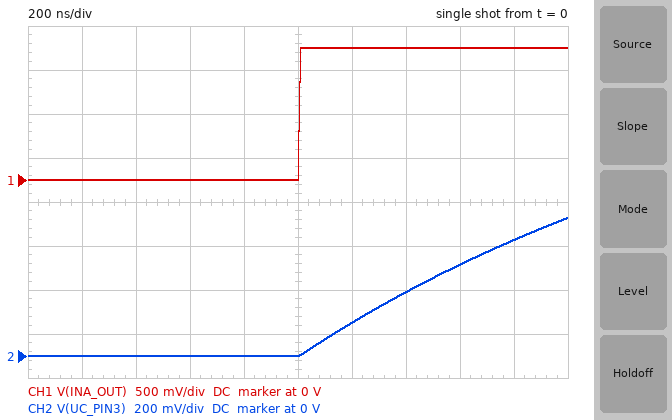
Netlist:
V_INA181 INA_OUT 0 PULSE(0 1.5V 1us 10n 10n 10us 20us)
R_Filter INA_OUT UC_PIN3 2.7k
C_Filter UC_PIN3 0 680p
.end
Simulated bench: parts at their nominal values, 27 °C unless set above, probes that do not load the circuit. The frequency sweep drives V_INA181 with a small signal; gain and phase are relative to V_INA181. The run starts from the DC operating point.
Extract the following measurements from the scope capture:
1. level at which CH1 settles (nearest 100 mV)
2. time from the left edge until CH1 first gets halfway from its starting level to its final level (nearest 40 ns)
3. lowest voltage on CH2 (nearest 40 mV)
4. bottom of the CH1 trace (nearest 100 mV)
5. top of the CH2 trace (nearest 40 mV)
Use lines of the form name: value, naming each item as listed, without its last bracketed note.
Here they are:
level at which CH1 settles: 1.5 V
time from the left edge until CH1 first gets halfway from its starting level to its final level: 1.00 µs
lowest voltage on CH2: 0 V
bottom of the CH1 trace: 0 V
top of the CH2 trace: 640 mV
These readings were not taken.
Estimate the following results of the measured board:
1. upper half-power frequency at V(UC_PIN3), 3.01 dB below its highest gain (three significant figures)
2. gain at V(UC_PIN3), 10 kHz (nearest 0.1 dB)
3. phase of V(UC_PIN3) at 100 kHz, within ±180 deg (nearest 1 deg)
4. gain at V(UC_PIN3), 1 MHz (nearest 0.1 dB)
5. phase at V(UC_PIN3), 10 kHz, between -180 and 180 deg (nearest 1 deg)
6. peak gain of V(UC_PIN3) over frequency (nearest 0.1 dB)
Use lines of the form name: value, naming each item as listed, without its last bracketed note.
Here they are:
upper half-power frequency at V(UC_PIN3), 3.01 dB below its highest gain: 86.7 kHz
gain at V(UC_PIN3), 10 kHz: -0.1 dB
phase of V(UC_PIN3) at 100 kHz, within ±180 deg: -49 deg
gain at V(UC_PIN3), 1 MHz: -21.3 dB
phase at V(UC_PIN3), 10 kHz, between -180 and 180 deg: -7 deg
peak gain of V(UC_PIN3) over frequency: 0 dB
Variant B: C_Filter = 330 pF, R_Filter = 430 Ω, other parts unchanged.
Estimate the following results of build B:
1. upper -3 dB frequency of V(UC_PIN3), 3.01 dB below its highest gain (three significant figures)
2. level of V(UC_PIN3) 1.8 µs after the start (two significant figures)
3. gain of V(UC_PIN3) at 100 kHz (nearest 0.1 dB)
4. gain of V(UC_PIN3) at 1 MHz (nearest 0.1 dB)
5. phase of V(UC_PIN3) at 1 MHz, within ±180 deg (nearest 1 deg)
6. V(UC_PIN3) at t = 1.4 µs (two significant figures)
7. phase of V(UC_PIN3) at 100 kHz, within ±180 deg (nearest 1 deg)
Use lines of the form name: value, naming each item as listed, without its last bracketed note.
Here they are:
upper -3 dB frequency of V(UC_PIN3), 3.01 dB below its highest gain: 1.12 MHz
level of V(UC_PIN3) 1.8 µs after the start: 1.5 V
gain of V(UC_PIN3) at 100 kHz: 0 dB
gain of V(UC_PIN3) at 1 MHz: -2.5 dB
phase of V(UC_PIN3) at 1 MHz, within ±180 deg: -42 deg
V(UC_PIN3) at t = 1.4 µs: 1.4 V
phase of V(UC_PIN3) at 100 kHz, within ±180 deg: -5 deg
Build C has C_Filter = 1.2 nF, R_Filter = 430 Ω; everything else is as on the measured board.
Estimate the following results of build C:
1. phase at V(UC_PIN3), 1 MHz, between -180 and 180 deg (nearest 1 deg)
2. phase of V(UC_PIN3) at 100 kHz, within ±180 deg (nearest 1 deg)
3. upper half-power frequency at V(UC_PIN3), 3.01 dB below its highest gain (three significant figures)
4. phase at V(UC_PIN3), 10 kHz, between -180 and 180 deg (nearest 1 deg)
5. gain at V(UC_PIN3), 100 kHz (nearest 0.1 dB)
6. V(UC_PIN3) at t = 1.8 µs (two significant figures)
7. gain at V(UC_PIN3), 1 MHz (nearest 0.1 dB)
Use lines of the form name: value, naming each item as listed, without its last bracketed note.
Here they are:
phase at V(UC_PIN3), 1 MHz, between -180 and 180 deg: -73 deg
phase of V(UC_PIN3) at 100 kHz, within ±180 deg: -18 deg
upper half-power frequency at V(UC_PIN3), 3.01 dB below its highest gain: 308 kHz
phase at V(UC_PIN3), 10 kHz, between -180 and 180 deg: -2 deg
gain at V(UC_PIN3), 100 kHz: -0.4 dB
V(UC_PIN3) at t = 1.8 µs: 1.2 V
gain at V(UC_PIN3), 1 MHz: -10.6 dB
